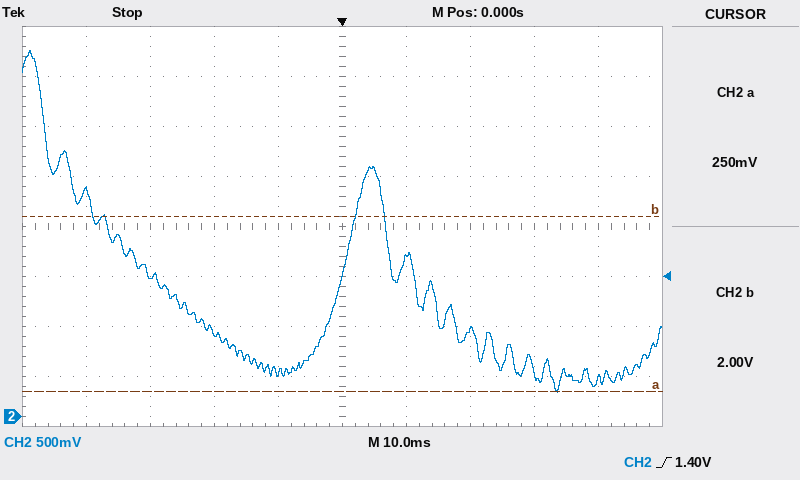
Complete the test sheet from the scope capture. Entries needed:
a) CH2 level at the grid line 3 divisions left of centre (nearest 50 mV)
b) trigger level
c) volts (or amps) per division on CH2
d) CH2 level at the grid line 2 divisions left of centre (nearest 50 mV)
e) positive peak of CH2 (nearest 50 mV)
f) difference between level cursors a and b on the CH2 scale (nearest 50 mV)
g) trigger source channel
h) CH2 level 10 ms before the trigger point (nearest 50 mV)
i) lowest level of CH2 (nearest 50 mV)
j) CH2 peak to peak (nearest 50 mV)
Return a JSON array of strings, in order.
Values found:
["1.40 V", "1.40 V", "500 mV", "850 mV", "3.65 V", "1.75 V", "CH2", "450 mV", "250 mV", "3.40 V"]
